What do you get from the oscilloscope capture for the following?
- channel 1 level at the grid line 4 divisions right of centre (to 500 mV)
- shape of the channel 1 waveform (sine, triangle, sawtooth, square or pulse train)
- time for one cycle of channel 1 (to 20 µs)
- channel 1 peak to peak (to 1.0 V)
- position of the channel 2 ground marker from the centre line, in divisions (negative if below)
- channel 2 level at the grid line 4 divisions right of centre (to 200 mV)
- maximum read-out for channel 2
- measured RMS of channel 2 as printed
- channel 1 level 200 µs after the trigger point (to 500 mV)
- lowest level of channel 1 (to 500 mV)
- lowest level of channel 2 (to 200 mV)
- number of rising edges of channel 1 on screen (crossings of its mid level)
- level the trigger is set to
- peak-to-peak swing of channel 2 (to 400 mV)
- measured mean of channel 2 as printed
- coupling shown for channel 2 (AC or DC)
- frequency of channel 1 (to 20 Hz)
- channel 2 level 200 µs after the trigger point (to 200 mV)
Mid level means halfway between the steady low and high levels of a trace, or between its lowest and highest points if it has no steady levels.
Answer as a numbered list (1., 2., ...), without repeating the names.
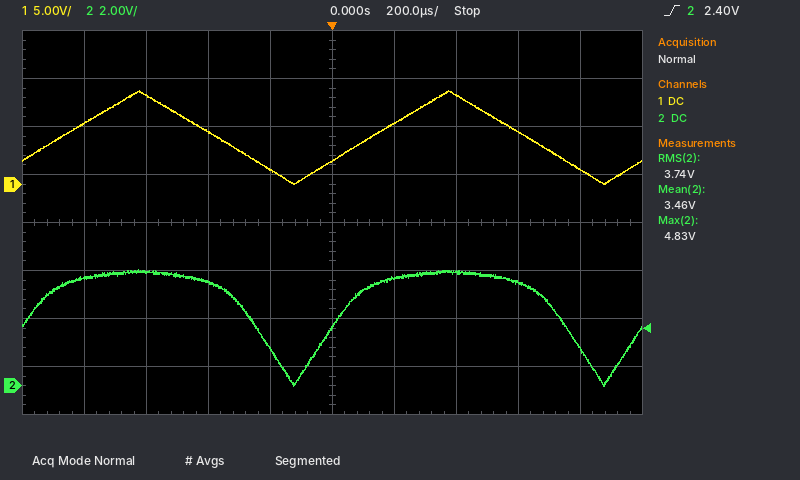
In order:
1. 1.5 V
2. triangle
3. 1.00 ms
4. 10.0 V
5. -3.4 div
6. 1.6 V
7. 4.83 V
8. 3.74 V
9. 6.5 V
10. 0.0 V
11. 0.0 V
12. 2
13. 2.40 V
14. 4.8 V
15. 3.46 V
16. DC
17. 1.00 kHz
18. 4.4 V
